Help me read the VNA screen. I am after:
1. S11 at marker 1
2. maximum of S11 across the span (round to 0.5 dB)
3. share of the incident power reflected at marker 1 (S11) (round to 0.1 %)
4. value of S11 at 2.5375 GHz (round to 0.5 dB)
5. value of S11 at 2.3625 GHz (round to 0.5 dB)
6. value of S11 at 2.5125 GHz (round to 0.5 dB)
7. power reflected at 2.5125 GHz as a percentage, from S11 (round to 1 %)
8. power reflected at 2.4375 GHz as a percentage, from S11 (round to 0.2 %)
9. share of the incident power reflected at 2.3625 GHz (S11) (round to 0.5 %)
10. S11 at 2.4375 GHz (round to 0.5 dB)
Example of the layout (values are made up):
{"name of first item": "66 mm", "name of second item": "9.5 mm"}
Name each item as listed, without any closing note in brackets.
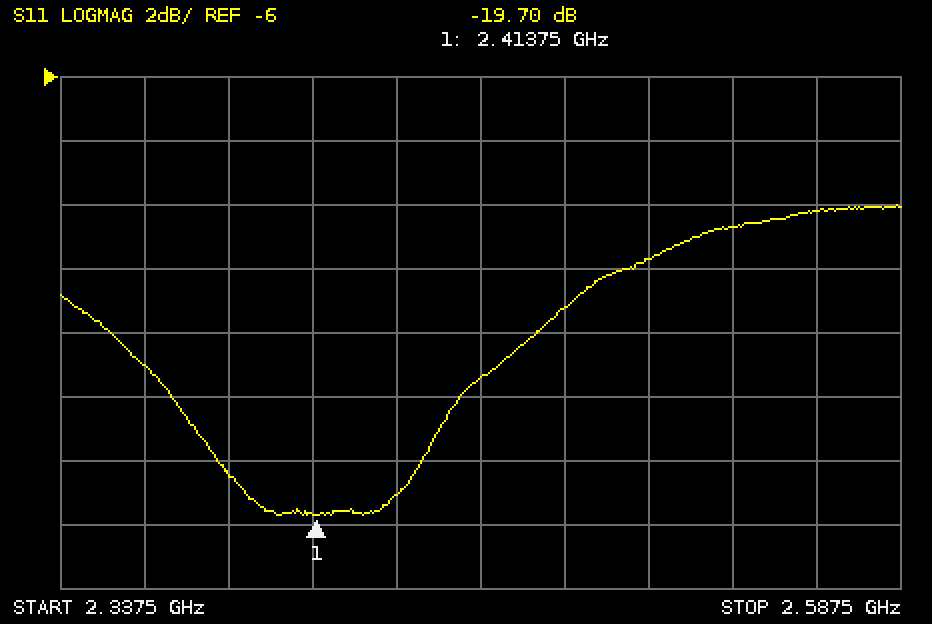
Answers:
{"S11 at marker 1": "-19.70 dB", "maximum of S11 across the span": "-10.0 dB", "share of the incident power reflected at marker 1 (S11)": "1.1 %", "value of S11 at 2.5375 GHz": "-10.5 dB", "value of S11 at 2.3625 GHz": "-15.0 dB", "value of S11 at 2.5125 GHz": "-11.5 dB", "power reflected at 2.5125 GHz as a percentage, from S11": "7 %", "power reflected at 2.4375 GHz as a percentage, from S11": "1.2 %", "share of the incident power reflected at 2.3625 GHz (S11)": "3.0 %", "S11 at 2.4375 GHz": "-19.0 dB"}
